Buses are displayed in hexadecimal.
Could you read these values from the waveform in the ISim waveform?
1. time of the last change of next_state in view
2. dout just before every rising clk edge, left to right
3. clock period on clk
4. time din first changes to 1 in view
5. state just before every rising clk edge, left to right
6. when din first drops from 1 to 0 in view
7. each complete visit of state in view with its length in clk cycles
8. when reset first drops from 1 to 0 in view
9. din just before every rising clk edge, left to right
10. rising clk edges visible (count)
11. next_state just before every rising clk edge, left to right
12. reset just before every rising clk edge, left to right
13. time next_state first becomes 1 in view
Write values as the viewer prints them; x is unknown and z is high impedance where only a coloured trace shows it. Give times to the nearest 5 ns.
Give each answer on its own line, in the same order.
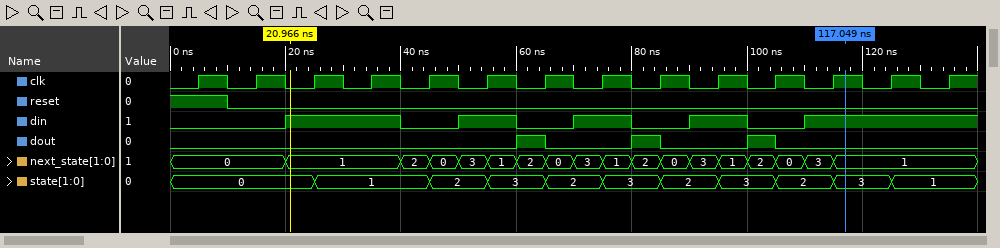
115 ns
0 0 0 0 0 0 1 0 1 0 1 0 0 0
10 ns
20 ns
0, 0, 0, 1, 1, 2, 3, 2, 3, 2, 3, 2, 3, 1
40 ns
1: 2, 2: 1, 3: 1, 2: 1, 3: 1, 2: 1, 3: 1, 2: 1, 3: 1
10 ns
0 0 1 1 0 1 0 1 0 1 0 1 1 1
14
0, 0, 1, 1, 2, 3, 2, 3, 2, 3, 2, 3, 1, 1
1 0 0 0 0 0 0 0 0 0 0 0 0 0
20 ns
